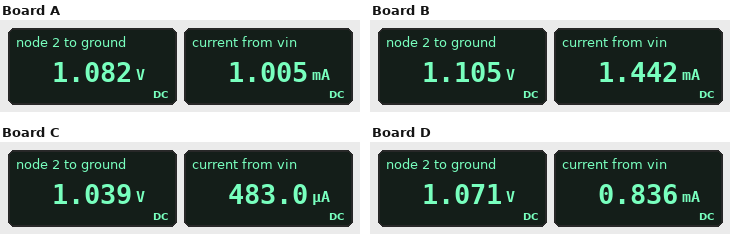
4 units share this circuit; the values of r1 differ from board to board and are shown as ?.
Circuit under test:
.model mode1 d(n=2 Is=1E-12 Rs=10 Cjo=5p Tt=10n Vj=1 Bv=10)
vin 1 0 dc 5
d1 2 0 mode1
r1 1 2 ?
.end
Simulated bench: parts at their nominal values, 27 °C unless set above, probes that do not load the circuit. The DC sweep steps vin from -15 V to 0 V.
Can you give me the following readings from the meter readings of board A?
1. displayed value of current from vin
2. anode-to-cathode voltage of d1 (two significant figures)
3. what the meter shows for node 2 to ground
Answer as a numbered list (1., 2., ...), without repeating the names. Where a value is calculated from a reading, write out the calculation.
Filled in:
1. 1.005 mA
2. 1.082 V = 1.1 V
3. 1.082 V
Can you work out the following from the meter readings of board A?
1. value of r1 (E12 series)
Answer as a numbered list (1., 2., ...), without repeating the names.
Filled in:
1. 3.9 kΩ
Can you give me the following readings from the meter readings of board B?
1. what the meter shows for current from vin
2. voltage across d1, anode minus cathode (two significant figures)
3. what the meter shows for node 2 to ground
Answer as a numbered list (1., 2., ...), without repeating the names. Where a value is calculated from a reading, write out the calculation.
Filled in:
1. 1.442 mA
2. 1.105 V = 1.1 V
3. 1.105 V
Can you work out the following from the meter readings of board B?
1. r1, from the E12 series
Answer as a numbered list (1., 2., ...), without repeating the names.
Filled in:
1. 2.7 kΩ
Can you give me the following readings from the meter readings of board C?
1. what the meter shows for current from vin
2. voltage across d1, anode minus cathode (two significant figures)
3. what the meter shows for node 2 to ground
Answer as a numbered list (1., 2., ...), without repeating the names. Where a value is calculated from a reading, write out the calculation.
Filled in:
1. 483.0 µA
2. 1.039 V = 1.0 V
3. 1.039 V
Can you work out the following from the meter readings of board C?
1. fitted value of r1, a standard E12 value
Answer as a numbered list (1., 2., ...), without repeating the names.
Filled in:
1. 8.2 kΩ
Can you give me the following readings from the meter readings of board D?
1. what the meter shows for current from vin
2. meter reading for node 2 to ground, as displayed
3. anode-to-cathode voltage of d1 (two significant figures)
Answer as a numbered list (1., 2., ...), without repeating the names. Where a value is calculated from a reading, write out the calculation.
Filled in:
1. 0.836 mA
2. 1.071 V
3. 1.071 V = 1.1 V
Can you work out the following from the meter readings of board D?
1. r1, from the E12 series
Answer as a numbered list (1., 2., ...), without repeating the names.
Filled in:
1. 4.7 kΩ
